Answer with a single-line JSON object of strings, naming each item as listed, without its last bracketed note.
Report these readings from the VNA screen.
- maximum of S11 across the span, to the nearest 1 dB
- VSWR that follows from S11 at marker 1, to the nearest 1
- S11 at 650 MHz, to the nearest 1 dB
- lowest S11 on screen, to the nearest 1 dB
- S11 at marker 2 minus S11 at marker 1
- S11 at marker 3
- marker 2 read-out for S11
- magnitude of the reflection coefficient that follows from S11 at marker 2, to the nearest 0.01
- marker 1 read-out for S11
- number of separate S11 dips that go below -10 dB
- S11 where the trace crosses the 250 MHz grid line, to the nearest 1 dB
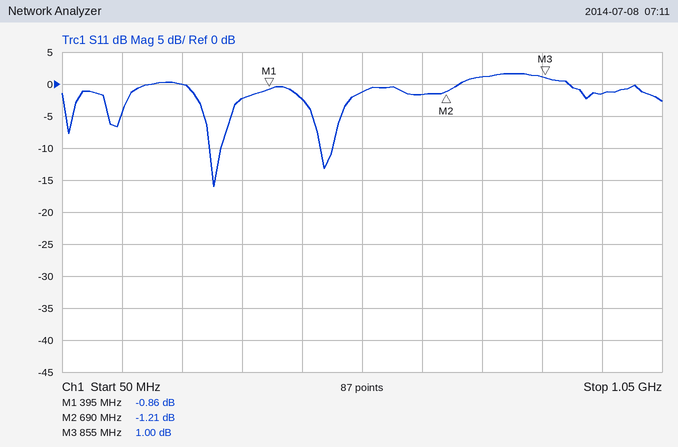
{"maximum of S11 across the span, to the nearest 1 dB": "2 dB", "VSWR that follows from S11 at marker 1, to the nearest 1": "20", "S11 at 650 MHz, to the nearest 1 dB": "-2 dB", "lowest S11 on screen, to the nearest 1 dB": "-16 dB", "S11 at marker 2 minus S11 at marker 1": "-0.35 dB", "S11 at marker 3": "1.00 dB", "marker 2 read-out for S11": "-1.21 dB", "magnitude of the reflection coefficient that follows from S11 at marker 2, to the nearest 0.01": "0.87", "marker 1 read-out for S11": "-0.86 dB", "number of separate S11 dips that go below -10 dB": "2", "S11 where the trace crosses the 250 MHz grid line, to the nearest 1 dB": "0 dB"}
